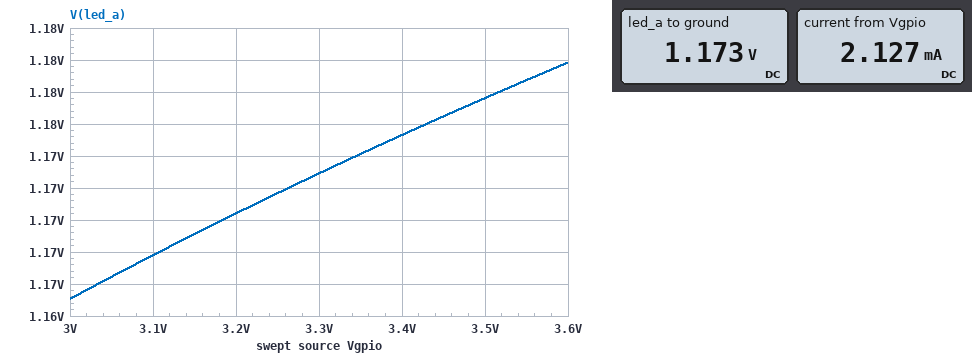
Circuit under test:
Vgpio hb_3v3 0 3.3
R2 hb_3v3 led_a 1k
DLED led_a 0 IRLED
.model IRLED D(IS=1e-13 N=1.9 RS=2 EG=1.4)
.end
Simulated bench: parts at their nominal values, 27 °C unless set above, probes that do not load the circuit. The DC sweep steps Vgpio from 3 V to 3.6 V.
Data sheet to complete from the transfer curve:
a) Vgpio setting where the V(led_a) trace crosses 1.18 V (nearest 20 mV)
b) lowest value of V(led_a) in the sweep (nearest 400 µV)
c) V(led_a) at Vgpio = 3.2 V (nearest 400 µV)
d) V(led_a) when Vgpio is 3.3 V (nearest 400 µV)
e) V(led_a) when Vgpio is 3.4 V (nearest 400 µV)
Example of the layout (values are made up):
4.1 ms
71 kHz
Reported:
3.52 V
1.1652 V
1.1704 V
1.1728 V
1.1752 V
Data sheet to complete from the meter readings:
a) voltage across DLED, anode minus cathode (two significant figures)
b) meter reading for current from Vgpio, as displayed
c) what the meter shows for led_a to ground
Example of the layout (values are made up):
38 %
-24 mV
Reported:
1.2 V
2.127 mA
1.173 V
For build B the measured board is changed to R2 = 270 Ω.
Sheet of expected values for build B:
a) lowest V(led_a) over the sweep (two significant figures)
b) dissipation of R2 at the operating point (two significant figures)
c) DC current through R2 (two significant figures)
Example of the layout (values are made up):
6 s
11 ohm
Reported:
1.2 V
16 mW
7.6 mA
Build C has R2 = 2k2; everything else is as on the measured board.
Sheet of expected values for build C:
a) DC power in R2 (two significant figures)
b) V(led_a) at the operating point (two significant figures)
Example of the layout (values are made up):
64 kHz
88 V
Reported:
2.1 mW
1.1 V
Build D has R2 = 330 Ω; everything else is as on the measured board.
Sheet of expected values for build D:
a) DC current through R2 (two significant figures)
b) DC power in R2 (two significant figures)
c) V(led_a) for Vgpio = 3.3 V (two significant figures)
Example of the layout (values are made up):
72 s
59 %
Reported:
6.3 mA
13 mW
1.2 V
